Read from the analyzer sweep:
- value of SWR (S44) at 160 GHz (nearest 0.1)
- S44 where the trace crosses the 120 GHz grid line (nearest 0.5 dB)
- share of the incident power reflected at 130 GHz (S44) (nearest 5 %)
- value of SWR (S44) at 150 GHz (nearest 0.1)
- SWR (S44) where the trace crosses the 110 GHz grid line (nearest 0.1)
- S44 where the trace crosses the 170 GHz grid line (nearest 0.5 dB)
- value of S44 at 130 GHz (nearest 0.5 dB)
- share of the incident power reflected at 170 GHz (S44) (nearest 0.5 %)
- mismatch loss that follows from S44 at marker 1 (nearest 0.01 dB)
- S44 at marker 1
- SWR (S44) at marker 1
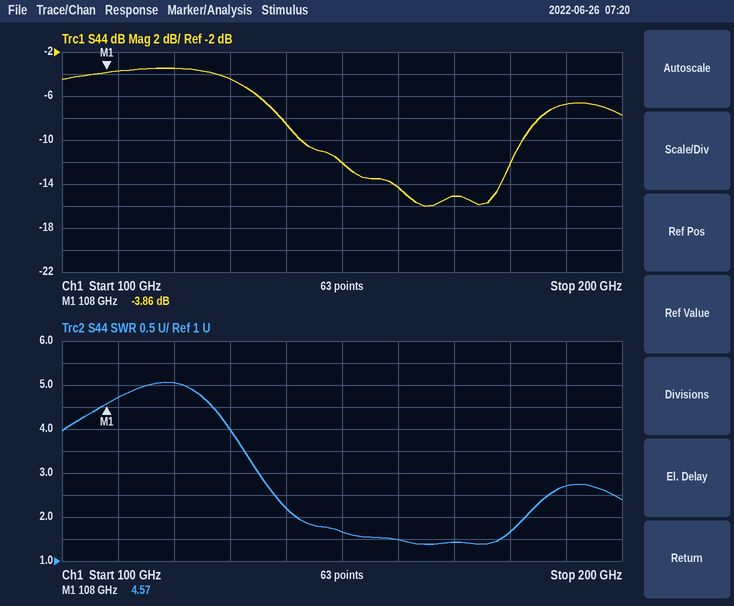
1.5
-3.5 dB
35 %
1.7
4.7
-15.0 dB
-4.5 dB
3.0 %
2.30 dB
-3.86 dB
4.57
